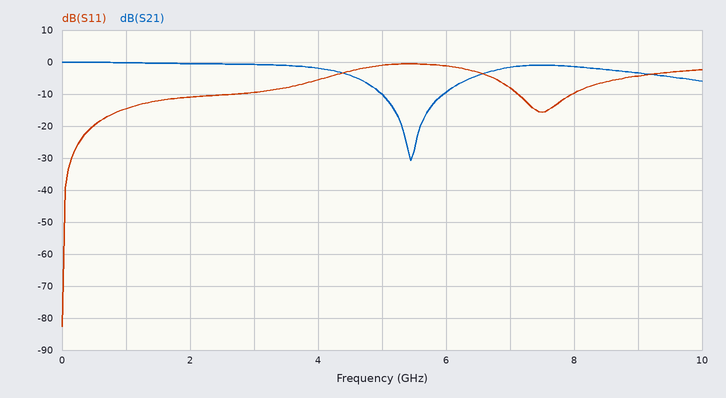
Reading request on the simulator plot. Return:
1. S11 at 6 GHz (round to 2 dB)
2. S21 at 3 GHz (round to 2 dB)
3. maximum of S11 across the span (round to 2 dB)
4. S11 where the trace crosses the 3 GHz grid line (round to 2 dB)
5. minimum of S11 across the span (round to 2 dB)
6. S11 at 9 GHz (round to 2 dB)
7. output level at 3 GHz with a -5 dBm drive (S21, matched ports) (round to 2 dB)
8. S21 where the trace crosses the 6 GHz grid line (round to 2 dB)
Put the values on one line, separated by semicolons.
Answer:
-2 dB; 0 dB; 0 dB; -10 dB; -82 dB; -4 dB; -6 dBm; -10 dB
